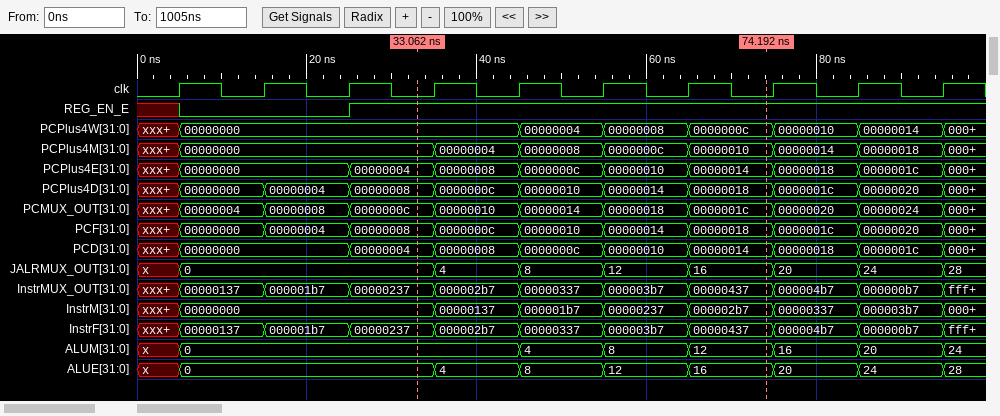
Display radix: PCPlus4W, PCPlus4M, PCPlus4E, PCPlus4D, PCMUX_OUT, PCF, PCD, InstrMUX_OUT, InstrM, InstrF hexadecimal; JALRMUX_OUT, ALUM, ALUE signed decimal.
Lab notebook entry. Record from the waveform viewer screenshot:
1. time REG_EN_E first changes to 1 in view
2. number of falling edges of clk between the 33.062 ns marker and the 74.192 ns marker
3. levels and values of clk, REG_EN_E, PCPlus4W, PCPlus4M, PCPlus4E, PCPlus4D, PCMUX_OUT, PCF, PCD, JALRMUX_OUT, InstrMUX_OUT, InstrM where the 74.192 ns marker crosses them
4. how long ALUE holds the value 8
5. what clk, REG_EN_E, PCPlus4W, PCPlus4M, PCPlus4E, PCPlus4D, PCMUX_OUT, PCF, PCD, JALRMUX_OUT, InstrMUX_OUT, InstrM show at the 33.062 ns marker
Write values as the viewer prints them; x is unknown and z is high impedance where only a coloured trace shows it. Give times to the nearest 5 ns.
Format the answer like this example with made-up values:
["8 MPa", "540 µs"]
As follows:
["25 ns", "4", "clk=0, REG_EN_E=1, PCPlus4W=0000000c, PCPlus4M=00000010, PCPlus4E=00000014, PCPlus4D=00000018, PCMUX_OUT=0000001c, PCF=00000018, PCD=00000014, JALRMUX_OUT=16, InstrMUX_OUT=00000437, InstrM=000002b7", "10 ns", "clk=0, REG_EN_E=1, PCPlus4W=00000000, PCPlus4M=00000000, PCPlus4E=00000004, PCPlus4D=00000008, PCMUX_OUT=0000000c, PCF=00000008, PCD=00000004, JALRMUX_OUT=0, InstrMUX_OUT=00000237, InstrM=00000000"]
